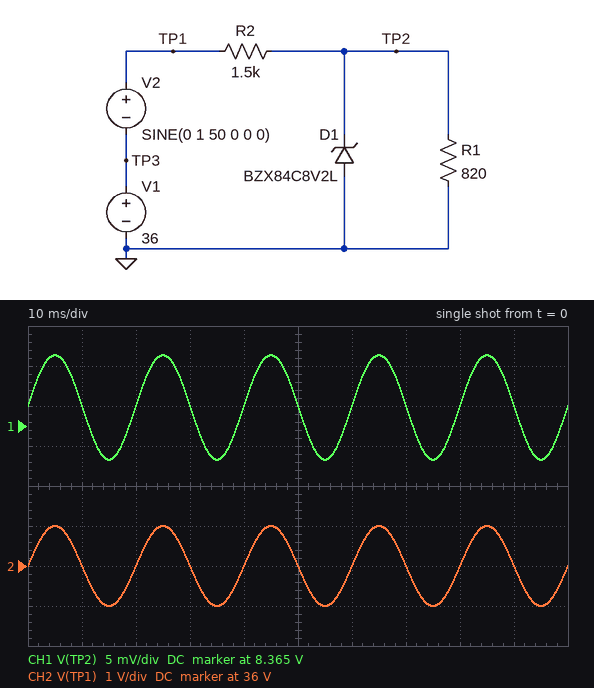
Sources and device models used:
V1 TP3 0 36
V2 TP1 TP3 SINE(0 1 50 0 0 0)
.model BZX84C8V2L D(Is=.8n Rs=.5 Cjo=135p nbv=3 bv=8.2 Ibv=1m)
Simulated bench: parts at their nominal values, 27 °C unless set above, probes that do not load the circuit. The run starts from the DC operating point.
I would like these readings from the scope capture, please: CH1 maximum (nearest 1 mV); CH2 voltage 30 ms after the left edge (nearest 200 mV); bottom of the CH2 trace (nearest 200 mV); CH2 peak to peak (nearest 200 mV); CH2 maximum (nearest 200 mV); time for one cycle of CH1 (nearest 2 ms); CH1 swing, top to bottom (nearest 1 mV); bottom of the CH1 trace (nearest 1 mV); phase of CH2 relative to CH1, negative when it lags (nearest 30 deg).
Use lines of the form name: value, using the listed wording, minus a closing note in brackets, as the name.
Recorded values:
CH1 maximum: 8.374 V
CH2 voltage 30 ms after the left edge: 36.0 V
bottom of the CH2 trace: 35.0 V
CH2 peak to peak: 2.0 V
CH2 maximum: 37.0 V
time for one cycle of CH1: 20 ms
CH1 swing, top to bottom: 13 mV
bottom of the CH1 trace: 8.361 V
phase of CH2 relative to CH1, negative when it lags: 0 deg
